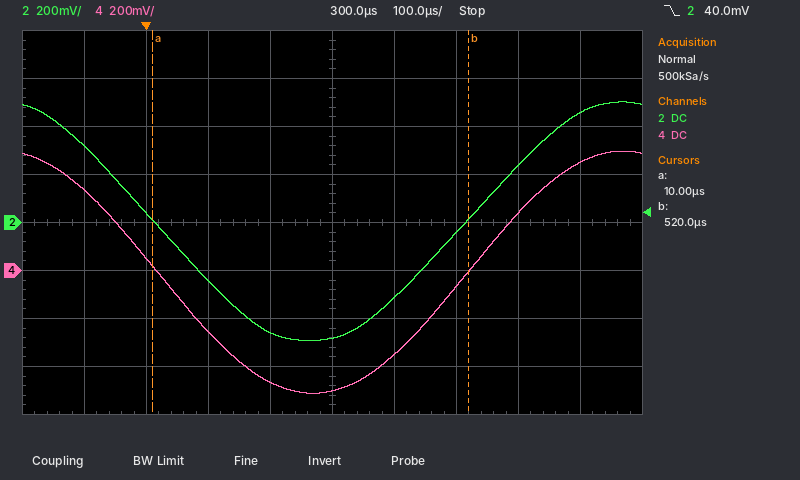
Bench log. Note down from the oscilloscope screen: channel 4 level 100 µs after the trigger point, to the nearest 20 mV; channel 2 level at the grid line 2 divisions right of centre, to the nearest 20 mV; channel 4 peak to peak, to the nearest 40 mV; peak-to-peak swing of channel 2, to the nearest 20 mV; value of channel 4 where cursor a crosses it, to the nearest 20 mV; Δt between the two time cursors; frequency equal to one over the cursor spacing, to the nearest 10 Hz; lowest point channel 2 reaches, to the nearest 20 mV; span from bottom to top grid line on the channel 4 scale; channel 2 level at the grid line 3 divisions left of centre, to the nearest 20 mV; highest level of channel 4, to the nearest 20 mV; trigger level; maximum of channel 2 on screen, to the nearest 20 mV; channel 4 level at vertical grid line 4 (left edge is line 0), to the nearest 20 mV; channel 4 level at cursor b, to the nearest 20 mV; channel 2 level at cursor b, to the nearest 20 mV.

-260 mV
-40 mV
1.00 V
1.00 V
20 mV
510 µs
1.96 kHz
-500 mV
1.6 V
40 mV
500 mV
40.0 mV
500 mV
-460 mV
0 mV
20 mV
